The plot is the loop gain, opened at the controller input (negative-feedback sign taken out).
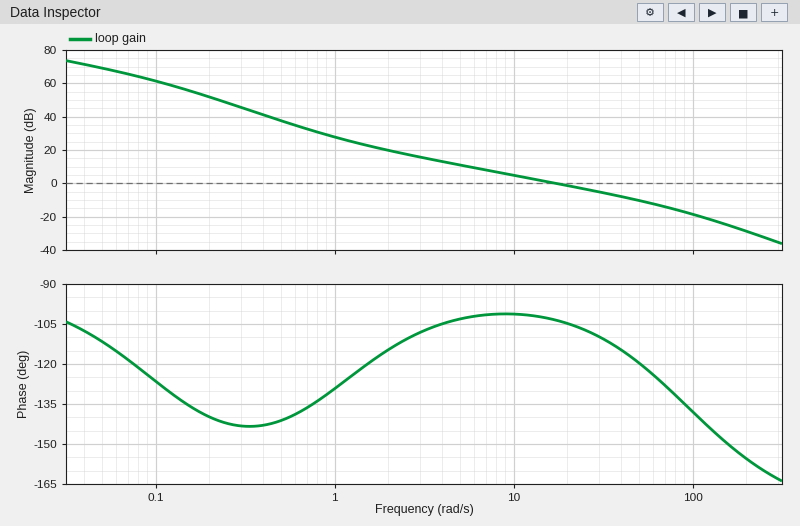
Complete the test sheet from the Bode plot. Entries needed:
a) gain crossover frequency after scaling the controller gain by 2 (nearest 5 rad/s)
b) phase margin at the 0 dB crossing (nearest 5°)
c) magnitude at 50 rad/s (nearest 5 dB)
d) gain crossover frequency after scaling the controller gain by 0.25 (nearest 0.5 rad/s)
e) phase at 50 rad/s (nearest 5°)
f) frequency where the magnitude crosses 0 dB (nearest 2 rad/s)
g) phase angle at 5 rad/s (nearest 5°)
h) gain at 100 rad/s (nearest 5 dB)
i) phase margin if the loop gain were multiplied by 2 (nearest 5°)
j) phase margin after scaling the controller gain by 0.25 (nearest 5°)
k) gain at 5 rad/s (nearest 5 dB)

35 rad/s
75°
-10 dB
4.5 rad/s
-120°
18 rad/s
-105°
-20 dB
70°
75°
10 dB
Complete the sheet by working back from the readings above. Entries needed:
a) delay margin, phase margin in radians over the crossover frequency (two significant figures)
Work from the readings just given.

0.073 s
